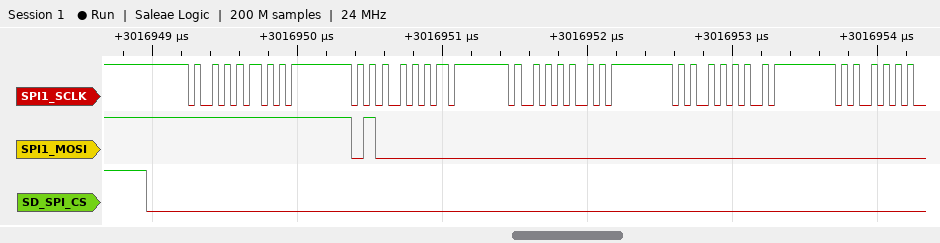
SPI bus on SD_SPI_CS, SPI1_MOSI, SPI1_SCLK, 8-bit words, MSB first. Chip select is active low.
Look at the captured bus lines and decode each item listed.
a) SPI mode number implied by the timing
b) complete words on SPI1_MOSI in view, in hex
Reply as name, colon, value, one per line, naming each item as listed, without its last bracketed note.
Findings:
SPI mode number implied by the timing: 3
complete words on SPI1_MOSI in view, in hex: FF, 40, 00, 00
